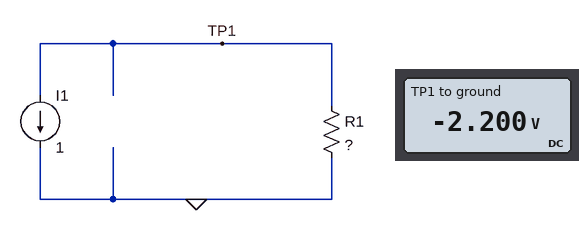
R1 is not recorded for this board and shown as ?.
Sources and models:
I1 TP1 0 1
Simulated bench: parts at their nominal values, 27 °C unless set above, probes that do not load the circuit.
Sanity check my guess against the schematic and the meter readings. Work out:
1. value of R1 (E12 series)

2.2 Ω
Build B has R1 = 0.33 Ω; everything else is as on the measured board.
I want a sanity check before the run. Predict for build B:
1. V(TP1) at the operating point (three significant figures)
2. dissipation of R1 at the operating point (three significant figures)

-330 mV
330 mW
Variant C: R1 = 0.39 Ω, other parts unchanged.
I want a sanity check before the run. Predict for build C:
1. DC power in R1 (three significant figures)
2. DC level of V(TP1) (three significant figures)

390 mW
-390 mV
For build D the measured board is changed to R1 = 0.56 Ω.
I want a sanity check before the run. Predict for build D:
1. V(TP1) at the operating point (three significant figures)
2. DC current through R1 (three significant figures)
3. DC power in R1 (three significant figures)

-560 mV
1.00 A
560 mW
